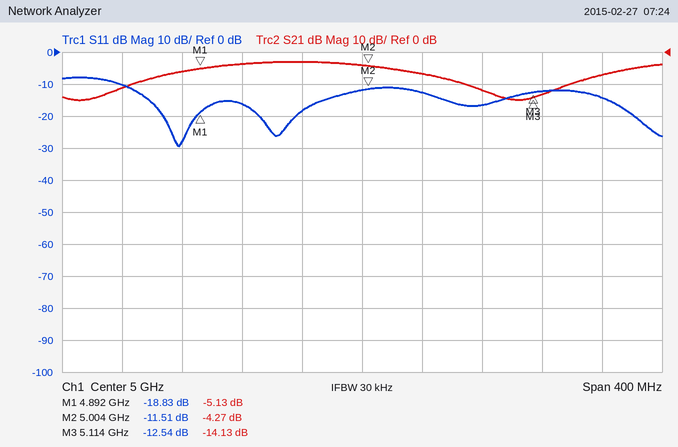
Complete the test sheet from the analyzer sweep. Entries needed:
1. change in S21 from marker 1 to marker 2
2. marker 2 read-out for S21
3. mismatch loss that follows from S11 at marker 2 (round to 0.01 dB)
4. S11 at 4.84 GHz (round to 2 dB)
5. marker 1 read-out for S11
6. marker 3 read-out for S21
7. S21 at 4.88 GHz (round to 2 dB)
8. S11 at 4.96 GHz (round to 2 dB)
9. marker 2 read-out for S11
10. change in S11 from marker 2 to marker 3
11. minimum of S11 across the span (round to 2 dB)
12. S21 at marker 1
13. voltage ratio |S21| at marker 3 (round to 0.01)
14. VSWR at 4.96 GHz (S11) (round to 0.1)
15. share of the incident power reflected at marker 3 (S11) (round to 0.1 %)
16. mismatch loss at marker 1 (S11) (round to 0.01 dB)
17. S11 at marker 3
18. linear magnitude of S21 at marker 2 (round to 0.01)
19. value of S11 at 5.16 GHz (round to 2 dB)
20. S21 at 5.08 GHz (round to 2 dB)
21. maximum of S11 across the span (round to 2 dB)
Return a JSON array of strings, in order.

["0.86 dB", "-4.27 dB", "0.32 dB", "-10 dB", "-18.83 dB", "-14.13 dB", "-6 dB", "-18 dB", "-11.51 dB", "-1.03 dB", "-30 dB", "-5.13 dB", "0.20", "1.3", "5.6 %", "0.06 dB", "-12.54 dB", "0.61", "-14 dB", "-12 dB", "-8 dB"]
